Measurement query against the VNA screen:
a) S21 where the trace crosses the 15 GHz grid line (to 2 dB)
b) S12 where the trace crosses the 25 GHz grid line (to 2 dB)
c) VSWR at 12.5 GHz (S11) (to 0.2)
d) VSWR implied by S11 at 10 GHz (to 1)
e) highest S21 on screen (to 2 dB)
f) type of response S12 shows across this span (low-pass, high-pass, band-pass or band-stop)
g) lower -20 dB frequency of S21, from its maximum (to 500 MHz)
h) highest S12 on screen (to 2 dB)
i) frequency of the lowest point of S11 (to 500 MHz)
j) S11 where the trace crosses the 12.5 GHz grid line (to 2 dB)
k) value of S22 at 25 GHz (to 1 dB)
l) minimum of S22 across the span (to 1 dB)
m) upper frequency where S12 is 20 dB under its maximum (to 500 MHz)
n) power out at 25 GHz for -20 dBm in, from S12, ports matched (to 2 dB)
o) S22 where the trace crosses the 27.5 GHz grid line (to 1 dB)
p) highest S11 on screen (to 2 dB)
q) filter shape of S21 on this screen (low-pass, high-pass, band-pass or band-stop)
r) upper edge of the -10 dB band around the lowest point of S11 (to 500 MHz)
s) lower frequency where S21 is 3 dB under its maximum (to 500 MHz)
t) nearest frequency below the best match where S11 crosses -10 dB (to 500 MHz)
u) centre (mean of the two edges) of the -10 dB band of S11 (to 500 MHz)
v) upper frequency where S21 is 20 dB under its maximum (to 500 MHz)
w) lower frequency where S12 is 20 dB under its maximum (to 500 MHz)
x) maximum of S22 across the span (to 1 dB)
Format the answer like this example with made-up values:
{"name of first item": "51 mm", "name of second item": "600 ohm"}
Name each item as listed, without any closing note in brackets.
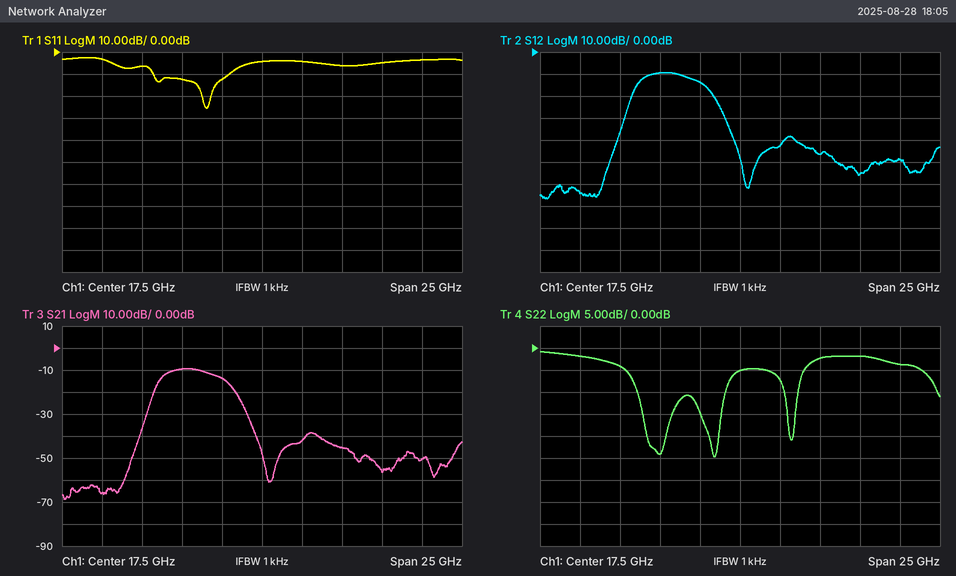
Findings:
{"S21 where the trace crosses the 15 GHz grid line": "-14 dB", "S12 where the trace crosses the 25 GHz grid line": "-56 dB", "VSWR at 12.5 GHz (S11)": "1.6", "VSWR implied by S11 at 10 GHz": "3", "highest S21 on screen": "-10 dB", "type of response S12 shows across this span": "band-pass", "lower -20 dB frequency of S21, from its maximum": "10.5 GHz", "highest S12 on screen": "-10 dB", "frequency of the lowest point of S11": "14.0 GHz", "S11 where the trace crosses the 12.5 GHz grid line": "-12 dB", "value of S22 at 25 GHz": "-2 dB", "minimum of S22 across the span": "-25 dB", "upper frequency where S12 is 20 dB under its maximum": "16.5 GHz", "power out at 25 GHz for -20 dBm in, from S12, ports matched": "-76 dBm", "S22 where the trace crosses the 27.5 GHz grid line": "-4 dB", "highest S11 on screen": "-2 dB", "filter shape of S21 on this screen": "band-pass", "upper edge of the -10 dB band around the lowest point of S11": "15.5 GHz", "lower frequency where S21 is 3 dB under its maximum": "11.5 GHz", "nearest frequency below the best match where S11 crosses -10 dB": "10.5 GHz", "centre (mean of the two edges) of the -10 dB band of S11": "13.0 GHz", "upper frequency where S21 is 20 dB under its maximum": "16.5 GHz", "lower frequency where S12 is 20 dB under its maximum": "10.5 GHz", "maximum of S22 across the span": "-1 dB"}
